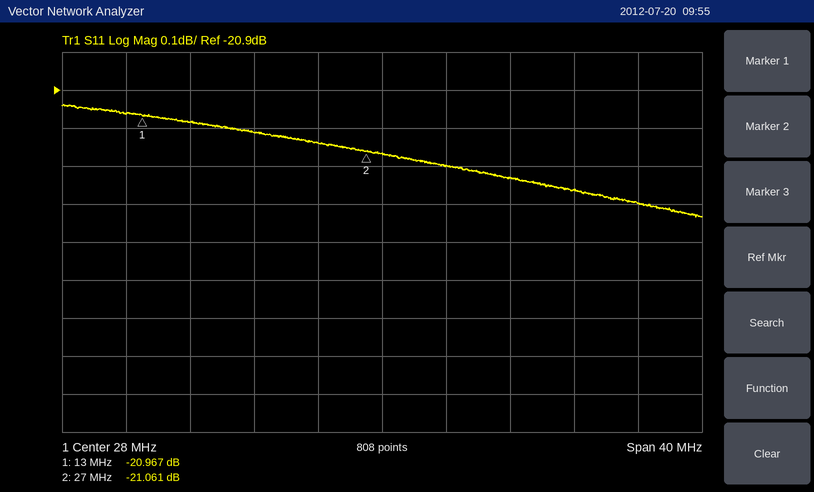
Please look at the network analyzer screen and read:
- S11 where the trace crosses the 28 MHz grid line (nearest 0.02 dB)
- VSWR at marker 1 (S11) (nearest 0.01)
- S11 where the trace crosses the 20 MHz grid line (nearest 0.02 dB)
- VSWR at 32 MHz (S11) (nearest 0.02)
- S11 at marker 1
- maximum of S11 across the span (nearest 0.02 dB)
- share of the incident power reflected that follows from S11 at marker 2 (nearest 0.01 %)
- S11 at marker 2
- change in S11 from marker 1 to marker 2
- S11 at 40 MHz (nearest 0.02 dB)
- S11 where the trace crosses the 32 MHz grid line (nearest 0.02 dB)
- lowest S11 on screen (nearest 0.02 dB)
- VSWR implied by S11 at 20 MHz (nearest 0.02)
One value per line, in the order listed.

-21.06 dB
1.20
-21.02 dB
1.20
-20.967 dB
-20.94 dB
0.78 %
-21.061 dB
-0.094 dB
-21.16 dB
-21.10 dB
-21.24 dB
1.20
